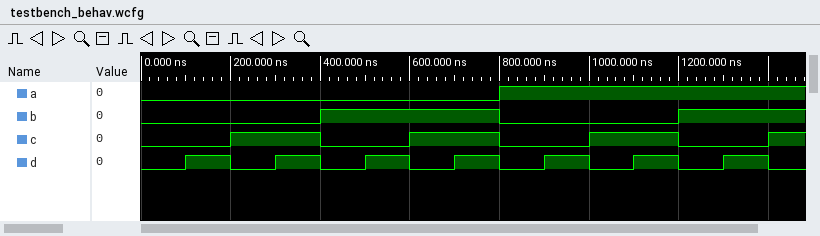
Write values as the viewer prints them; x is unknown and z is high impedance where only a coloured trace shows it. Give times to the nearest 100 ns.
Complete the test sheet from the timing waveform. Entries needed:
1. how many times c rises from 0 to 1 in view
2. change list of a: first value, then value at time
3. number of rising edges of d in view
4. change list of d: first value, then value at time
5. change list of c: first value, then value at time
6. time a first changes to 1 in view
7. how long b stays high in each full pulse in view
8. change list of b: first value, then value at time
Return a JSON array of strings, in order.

["4", "0, 1 at 800 ns", "7", "0, 1 at 100 ns, 0 at 200 ns, 1 at 300 ns, 0 at 400 ns, 1 at 500 ns, 0 at 600 ns, 1 at 700 ns, 0 at 800 ns, 1 at 900 ns, 0 at 1000 ns, 1 at 1100 ns, 0 at 1200 ns, 1 at 1300 ns, 0 at 1400 ns", "0, 1 at 200 ns, 0 at 400 ns, 1 at 600 ns, 0 at 800 ns, 1 at 1000 ns, 0 at 1200 ns, 1 at 1400 ns", "800 ns", "400 ns", "0, 1 at 400 ns, 0 at 800 ns, 1 at 1200 ns"]
